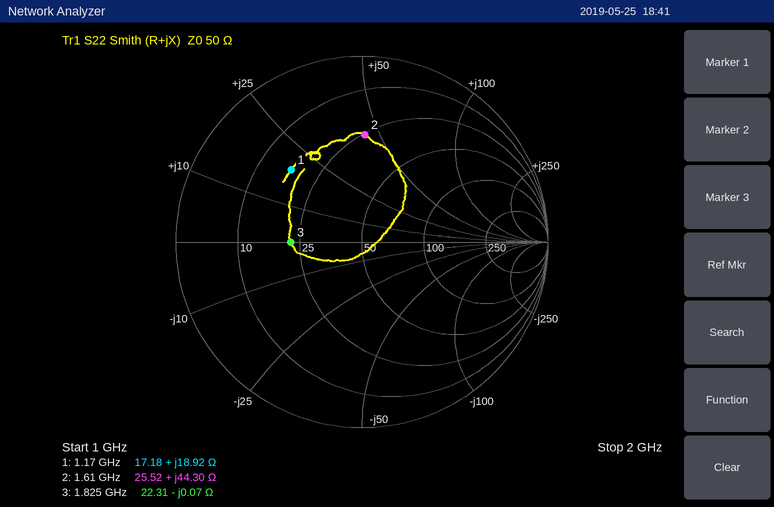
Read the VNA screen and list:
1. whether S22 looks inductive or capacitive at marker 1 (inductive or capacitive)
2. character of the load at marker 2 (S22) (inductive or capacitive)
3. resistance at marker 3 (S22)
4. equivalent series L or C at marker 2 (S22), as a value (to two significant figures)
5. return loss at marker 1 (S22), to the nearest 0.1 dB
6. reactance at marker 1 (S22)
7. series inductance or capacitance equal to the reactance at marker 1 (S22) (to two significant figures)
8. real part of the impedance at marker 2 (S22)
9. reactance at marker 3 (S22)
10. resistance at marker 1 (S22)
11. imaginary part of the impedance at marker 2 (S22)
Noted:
inductive
inductive
22.31 Ω
4.4 nH
5.3 dB
+18.92 Ω
2.6 nH
25.52 Ω
-0.07 Ω
17.18 Ω
+44.30 Ω
